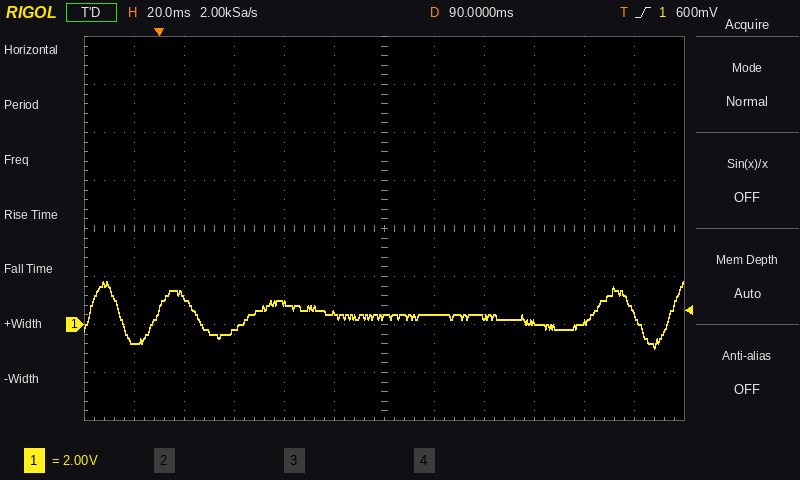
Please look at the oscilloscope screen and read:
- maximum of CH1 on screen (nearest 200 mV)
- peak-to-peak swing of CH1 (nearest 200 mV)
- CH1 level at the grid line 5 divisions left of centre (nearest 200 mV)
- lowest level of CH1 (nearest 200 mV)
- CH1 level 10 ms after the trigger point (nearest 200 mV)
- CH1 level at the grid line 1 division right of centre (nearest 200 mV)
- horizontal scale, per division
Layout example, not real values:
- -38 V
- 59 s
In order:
- 1.8 V
- 2.8 V
- -800 mV
- -1.0 V
- 1.2 V
- 400 mV
- 20 ms
